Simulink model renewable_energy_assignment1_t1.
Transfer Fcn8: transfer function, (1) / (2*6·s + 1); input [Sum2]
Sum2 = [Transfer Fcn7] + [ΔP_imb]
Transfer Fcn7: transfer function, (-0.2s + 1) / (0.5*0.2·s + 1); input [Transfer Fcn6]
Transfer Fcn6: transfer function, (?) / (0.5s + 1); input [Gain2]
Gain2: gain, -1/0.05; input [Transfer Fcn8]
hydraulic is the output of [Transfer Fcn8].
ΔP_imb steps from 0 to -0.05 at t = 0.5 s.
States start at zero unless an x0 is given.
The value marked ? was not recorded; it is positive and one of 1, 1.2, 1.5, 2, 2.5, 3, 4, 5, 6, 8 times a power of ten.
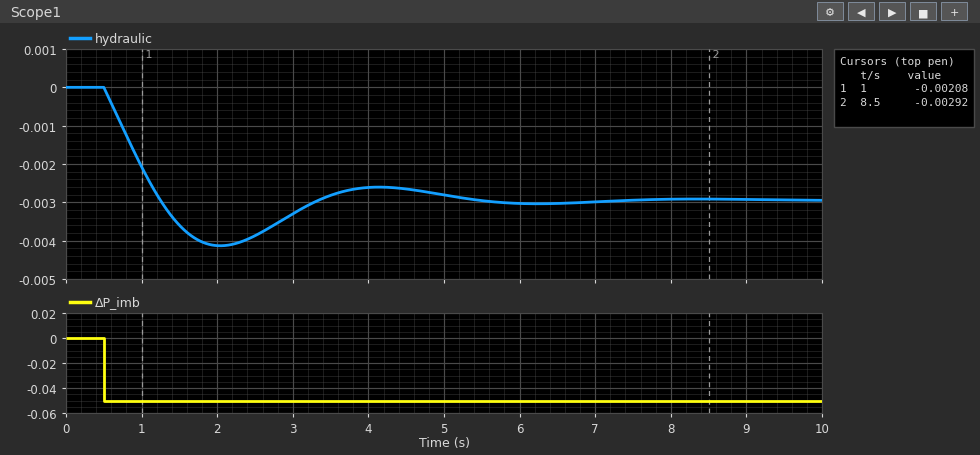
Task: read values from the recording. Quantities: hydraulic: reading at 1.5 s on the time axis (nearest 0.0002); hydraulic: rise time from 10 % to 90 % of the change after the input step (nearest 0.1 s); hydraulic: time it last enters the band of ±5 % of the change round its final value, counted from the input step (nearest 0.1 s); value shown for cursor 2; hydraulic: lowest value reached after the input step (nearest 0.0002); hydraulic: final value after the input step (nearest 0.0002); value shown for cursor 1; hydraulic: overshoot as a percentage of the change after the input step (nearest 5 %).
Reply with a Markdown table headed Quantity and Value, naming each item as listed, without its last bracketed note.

| Quantity | Value |
|---|---|
| hydraulic: reading at 1.5 s on the time axis | -0.0036 |
| hydraulic: rise time from 10 % to 90 % of the change after the input step | 0.6 s |
| hydraulic: time it last enters the band of ±5 % of the change round its final value, counted from the input step | 4.5 s |
| value shown for cursor 2 | -0.00292 |
| hydraulic: lowest value reached after the input step | -0.0042 |
| hydraulic: final value after the input step | -0.0030 |
| value shown for cursor 1 | -0.00208 |
| hydraulic: overshoot as a percentage of the change after the input step | 40 % |
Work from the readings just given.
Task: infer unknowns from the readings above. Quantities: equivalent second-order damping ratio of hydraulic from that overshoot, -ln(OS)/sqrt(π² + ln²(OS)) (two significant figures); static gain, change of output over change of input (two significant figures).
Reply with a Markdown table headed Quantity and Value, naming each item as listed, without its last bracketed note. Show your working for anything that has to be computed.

| Quantity | Value |
|---|---|
| equivalent second-order damping ratio of hydraulic from that overshoot, -ln(OS)/sqrt(π² + ln²(OS)) | ln(0.4) = -0.916; 0.916 / sqrt(9.870 + 0.840) = 0.28 |
| static gain, change of output over change of input | (-0.003 - 0) / (-0.05 - 0) = 0.060 |
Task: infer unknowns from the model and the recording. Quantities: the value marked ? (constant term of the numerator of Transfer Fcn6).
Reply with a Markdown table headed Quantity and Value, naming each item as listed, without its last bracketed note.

| Quantity | Value |
|---|---|
| the value marked ? | 0.8 |
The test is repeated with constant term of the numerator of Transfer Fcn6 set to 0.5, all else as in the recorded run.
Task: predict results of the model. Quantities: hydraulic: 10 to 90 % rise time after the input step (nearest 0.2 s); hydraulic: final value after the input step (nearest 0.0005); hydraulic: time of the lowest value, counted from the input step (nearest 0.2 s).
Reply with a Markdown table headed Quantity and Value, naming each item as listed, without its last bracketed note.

| Quantity | Value |
|---|---|
| hydraulic: 10 to 90 % rise time after the input step | 1.0 s |
| hydraulic: final value after the input step | -0.0045 |
| hydraulic: time of the lowest value, counted from the input step | 2.2 s |
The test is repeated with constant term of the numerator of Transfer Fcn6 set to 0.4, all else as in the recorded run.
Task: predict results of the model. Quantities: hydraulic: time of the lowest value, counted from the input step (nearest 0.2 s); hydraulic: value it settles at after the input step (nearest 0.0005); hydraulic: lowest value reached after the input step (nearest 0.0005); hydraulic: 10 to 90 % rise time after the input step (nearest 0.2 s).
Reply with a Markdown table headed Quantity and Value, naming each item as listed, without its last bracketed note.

| Quantity | Value |
|---|---|
| hydraulic: time of the lowest value, counted from the input step | 2.8 s |
| hydraulic: value it settles at after the input step | -0.0055 |
| hydraulic: lowest value reached after the input step | -0.0060 |
| hydraulic: 10 to 90 % rise time after the input step | 1.4 s |
